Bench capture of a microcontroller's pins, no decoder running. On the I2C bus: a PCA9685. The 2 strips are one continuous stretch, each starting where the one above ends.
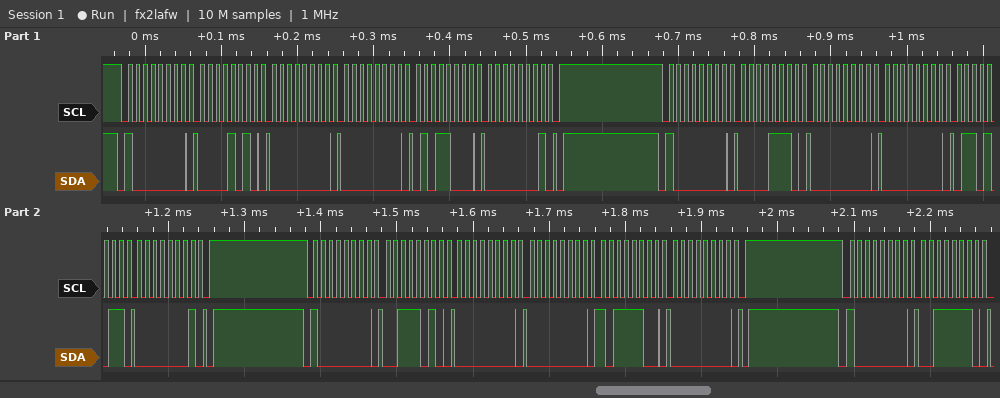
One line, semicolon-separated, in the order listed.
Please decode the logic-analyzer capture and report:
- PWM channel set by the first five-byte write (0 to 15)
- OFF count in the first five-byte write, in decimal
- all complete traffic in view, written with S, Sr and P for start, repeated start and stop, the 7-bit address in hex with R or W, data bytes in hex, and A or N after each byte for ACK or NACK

1; 344; S 40W A 0A A 00 A 00 A 58 A 01 A P S 40W A 0E A 00 A 00 A 6B A 01 A P S 40W A 3A A 00 A 00 A BC A 00 A P S 40W A 3E A
